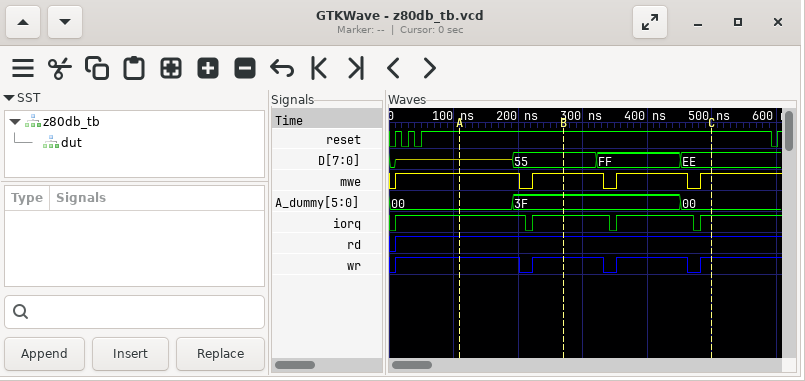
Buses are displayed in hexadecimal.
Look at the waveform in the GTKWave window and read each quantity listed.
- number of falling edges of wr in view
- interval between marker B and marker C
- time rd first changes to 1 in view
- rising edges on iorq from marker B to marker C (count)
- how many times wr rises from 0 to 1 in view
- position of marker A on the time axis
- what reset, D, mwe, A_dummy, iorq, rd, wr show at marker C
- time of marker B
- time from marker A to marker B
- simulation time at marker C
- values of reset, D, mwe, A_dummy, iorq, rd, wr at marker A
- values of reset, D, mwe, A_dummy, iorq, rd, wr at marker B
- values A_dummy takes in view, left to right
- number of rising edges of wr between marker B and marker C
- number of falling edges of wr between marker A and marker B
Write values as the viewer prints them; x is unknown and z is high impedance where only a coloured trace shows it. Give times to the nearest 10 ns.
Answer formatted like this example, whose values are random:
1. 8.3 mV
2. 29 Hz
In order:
1. 3
2. 230 ns
3. 10 ns
4. 2
5. 4
6. 110 ns
7. reset=1, D=EE, mwe=1, A_dummy=00, iorq=1, rd=1, wr=1
8. 270 ns
9. 160 ns
10. 500 ns
11. reset=1, D=z, mwe=1, A_dummy=00, iorq=1, rd=1, wr=1
12. reset=1, D=55, mwe=1, A_dummy=3F, iorq=1, rd=1, wr=1
13. 00, 3F, 00
14. 2
15. 1
